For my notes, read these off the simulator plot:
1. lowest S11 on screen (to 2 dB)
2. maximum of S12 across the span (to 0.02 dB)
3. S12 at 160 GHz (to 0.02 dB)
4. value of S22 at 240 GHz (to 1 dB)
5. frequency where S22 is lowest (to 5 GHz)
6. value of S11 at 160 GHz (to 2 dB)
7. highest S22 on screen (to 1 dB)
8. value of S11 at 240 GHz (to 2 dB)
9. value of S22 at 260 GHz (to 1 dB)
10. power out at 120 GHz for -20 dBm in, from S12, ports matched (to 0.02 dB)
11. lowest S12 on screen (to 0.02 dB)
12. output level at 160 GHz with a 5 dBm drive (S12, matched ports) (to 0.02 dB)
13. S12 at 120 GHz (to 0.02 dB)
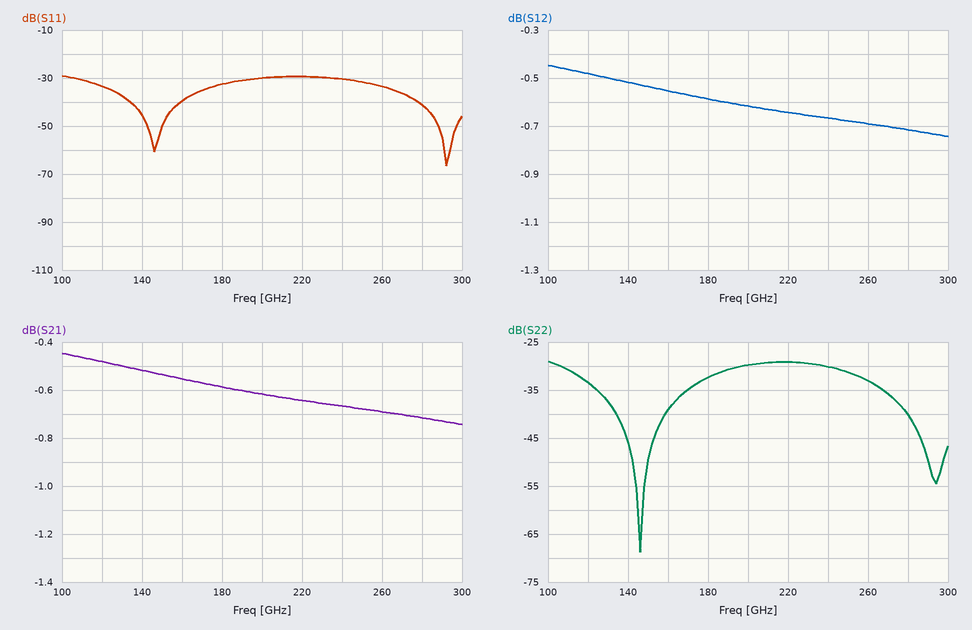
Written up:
-66 dB
-0.44 dB
-0.56 dB
-30 dB
145 GHz
-40 dB
-29 dB
-30 dB
-33 dB
-20.48 dBm
-0.74 dB
4.44 dBm
-0.48 dB
